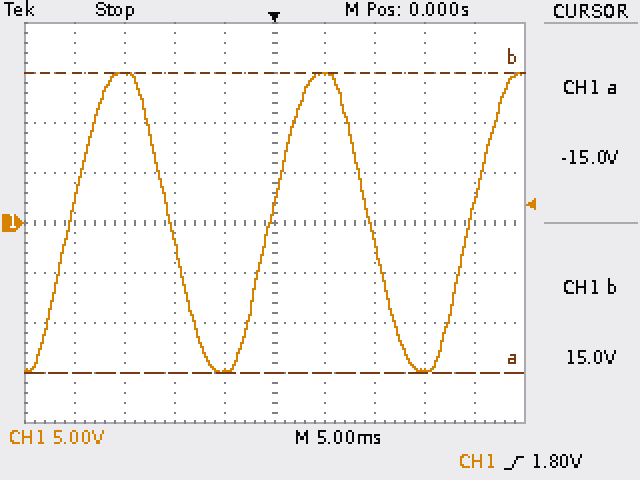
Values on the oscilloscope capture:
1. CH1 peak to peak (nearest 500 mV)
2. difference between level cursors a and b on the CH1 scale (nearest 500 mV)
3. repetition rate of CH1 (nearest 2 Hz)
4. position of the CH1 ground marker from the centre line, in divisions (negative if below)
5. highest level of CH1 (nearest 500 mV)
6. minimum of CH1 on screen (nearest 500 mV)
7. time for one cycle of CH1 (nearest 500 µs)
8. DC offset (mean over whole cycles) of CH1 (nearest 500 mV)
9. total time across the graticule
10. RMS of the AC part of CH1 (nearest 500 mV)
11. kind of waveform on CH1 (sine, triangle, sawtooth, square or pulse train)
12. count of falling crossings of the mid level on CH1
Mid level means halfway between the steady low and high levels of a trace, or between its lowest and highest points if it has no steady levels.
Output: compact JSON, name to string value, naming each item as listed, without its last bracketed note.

{"CH1 peak to peak": "30.0 V", "difference between level cursors a and b on the CH1 scale": "30.0 V", "repetition rate of CH1": "50 Hz", "position of the CH1 ground marker from the centre line, in divisions": "0.0 div", "highest level of CH1": "15.0 V", "minimum of CH1 on screen": "-15.0 V", "time for one cycle of CH1": "20.0 ms", "DC offset (mean over whole cycles) of CH1": "0.0 V", "total time across the graticule": "50 ms", "RMS of the AC part of CH1": "10.5 V", "kind of waveform on CH1": "sine", "count of falling crossings of the mid level on CH1": "2"}
